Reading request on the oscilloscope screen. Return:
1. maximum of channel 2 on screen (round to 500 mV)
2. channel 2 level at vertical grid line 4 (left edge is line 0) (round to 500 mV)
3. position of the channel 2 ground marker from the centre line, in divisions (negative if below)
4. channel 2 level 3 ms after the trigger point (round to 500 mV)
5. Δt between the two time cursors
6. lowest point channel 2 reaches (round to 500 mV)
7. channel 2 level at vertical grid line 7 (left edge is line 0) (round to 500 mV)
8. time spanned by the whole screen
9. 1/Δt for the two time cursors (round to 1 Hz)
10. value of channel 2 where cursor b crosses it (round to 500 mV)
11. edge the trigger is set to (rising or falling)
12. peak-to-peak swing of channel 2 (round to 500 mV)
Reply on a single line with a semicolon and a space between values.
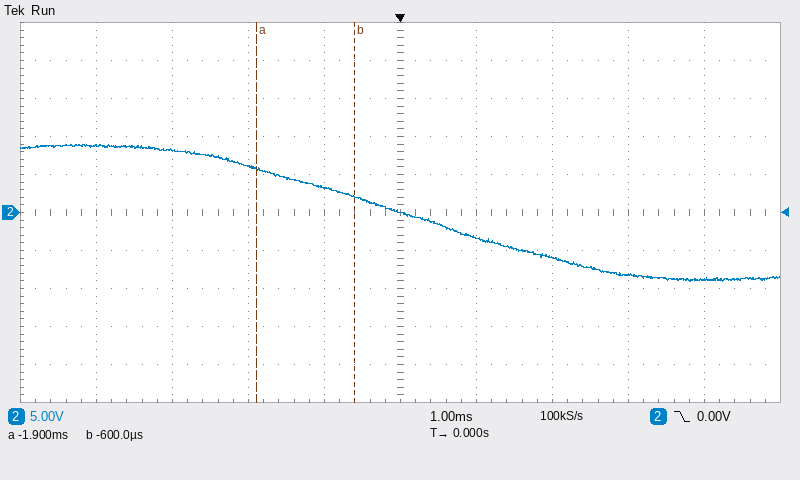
9.0 V; 3.5 V; 0.0 div; -8.0 V; 1.3 ms; -9.0 V; -6.0 V; 10 ms; 769 Hz; 2.0 V; falling; 18.0 V
